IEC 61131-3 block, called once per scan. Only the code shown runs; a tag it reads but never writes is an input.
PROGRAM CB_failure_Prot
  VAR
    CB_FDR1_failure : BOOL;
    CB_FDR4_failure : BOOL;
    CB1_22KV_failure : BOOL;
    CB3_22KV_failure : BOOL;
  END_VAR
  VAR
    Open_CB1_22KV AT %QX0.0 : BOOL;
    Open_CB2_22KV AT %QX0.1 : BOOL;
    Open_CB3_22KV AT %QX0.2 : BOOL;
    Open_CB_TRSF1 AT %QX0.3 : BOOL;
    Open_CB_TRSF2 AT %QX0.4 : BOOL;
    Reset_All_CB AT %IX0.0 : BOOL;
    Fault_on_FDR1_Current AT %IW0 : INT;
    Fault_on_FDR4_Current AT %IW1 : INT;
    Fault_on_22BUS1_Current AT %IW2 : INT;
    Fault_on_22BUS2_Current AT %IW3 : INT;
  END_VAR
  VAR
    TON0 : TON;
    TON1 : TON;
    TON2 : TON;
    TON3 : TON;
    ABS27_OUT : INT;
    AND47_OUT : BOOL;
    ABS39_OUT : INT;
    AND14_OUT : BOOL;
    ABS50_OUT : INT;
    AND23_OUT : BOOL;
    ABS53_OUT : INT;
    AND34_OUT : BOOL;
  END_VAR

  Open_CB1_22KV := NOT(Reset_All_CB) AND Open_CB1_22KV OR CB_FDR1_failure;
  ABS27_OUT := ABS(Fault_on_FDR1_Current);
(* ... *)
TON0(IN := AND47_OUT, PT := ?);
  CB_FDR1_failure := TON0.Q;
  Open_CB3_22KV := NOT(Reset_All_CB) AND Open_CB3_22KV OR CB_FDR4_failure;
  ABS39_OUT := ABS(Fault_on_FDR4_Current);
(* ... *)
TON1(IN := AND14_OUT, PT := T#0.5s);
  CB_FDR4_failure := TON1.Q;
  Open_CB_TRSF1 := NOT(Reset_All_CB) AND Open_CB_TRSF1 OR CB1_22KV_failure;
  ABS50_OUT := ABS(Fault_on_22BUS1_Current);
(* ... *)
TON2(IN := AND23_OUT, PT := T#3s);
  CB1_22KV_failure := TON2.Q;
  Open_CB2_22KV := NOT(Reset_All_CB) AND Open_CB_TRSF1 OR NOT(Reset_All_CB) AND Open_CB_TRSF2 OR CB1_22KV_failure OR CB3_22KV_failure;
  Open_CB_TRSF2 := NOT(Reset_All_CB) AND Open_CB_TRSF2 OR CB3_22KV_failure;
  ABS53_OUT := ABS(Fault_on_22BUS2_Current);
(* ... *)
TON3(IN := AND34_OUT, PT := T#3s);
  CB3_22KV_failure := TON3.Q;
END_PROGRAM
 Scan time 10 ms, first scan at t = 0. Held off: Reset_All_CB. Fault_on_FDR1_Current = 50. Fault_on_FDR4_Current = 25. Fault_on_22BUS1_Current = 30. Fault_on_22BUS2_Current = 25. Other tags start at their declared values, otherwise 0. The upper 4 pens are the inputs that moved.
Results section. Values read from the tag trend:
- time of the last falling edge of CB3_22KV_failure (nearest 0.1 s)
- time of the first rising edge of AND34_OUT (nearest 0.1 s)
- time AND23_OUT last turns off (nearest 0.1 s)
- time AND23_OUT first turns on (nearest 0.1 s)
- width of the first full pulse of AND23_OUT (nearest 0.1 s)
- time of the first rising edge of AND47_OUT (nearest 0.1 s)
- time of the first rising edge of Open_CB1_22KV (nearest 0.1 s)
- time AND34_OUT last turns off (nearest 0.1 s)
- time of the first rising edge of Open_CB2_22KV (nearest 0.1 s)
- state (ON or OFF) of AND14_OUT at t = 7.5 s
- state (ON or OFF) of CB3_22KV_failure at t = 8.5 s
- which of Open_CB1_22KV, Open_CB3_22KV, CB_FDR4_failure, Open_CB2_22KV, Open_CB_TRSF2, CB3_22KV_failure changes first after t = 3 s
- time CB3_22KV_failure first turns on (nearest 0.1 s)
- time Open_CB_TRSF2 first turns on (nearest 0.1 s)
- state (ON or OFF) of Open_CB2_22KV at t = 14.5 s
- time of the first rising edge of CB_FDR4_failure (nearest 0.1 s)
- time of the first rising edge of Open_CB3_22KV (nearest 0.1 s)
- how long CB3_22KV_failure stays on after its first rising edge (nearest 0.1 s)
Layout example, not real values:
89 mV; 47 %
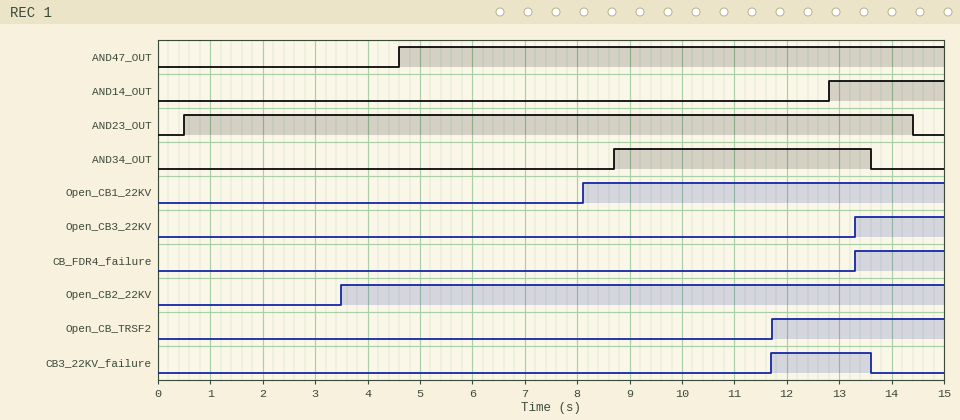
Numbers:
13.6 s; 8.7 s; 14.4 s; 0.5 s; 13.9 s; 4.6 s; 8.1 s; 13.6 s; 3.5 s; OFF; OFF; Open_CB2_22KV; 11.7 s; 11.7 s; ON; 13.3 s; 13.3 s; 1.9 s
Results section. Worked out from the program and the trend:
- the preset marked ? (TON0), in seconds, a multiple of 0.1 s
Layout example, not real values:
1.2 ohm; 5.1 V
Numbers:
3.5 s
